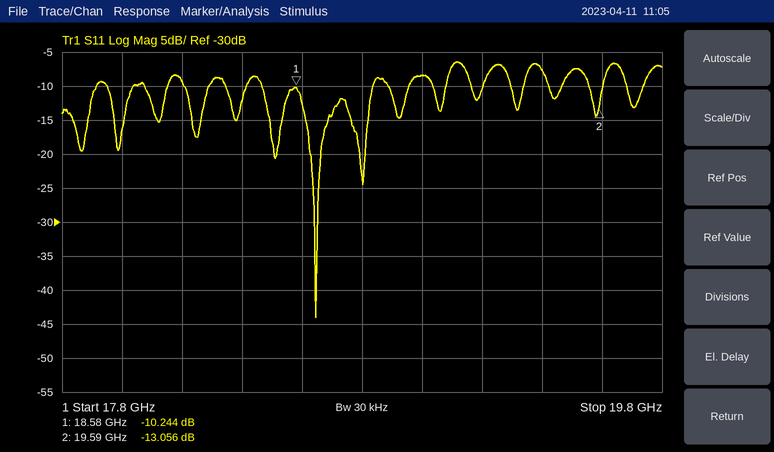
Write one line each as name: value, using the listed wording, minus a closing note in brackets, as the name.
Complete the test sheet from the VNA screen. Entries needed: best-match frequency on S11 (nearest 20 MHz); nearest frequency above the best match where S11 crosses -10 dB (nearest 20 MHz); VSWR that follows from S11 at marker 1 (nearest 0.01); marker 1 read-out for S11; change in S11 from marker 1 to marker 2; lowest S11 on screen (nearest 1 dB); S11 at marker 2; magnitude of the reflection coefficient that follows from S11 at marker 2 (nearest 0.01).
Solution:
best-match frequency on S11: 18.64 GHz
nearest frequency above the best match where S11 crosses -10 dB: 18.84 GHz
VSWR that follows from S11 at marker 1: 1.89
marker 1 read-out for S11: -10.244 dB
change in S11 from marker 1 to marker 2: -2.812 dB
lowest S11 on screen: -44 dB
S11 at marker 2: -13.056 dB
magnitude of the reflection coefficient that follows from S11 at marker 2: 0.22
